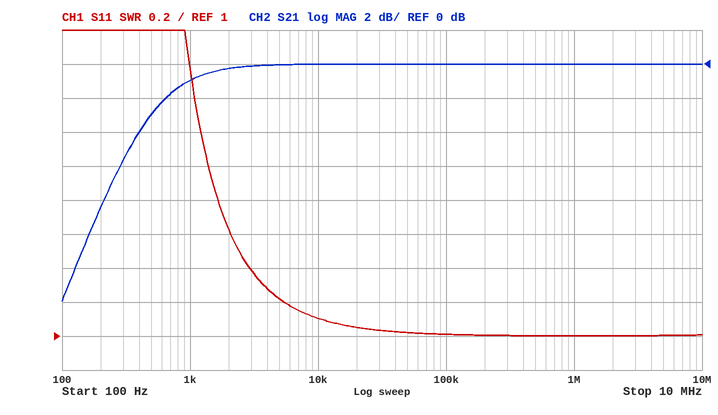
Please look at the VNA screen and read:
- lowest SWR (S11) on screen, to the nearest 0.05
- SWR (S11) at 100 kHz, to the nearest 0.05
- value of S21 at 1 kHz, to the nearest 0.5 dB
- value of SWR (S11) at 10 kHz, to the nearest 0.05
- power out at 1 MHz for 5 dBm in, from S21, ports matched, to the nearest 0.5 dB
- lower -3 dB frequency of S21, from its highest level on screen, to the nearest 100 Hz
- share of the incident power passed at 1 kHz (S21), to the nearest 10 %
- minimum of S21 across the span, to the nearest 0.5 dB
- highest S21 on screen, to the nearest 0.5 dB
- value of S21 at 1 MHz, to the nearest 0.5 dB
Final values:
1.00
1.00
-1.0 dB
1.10
5.0 dBm
500 Hz
80 %
-14.0 dB
0.0 dB
0.0 dB
